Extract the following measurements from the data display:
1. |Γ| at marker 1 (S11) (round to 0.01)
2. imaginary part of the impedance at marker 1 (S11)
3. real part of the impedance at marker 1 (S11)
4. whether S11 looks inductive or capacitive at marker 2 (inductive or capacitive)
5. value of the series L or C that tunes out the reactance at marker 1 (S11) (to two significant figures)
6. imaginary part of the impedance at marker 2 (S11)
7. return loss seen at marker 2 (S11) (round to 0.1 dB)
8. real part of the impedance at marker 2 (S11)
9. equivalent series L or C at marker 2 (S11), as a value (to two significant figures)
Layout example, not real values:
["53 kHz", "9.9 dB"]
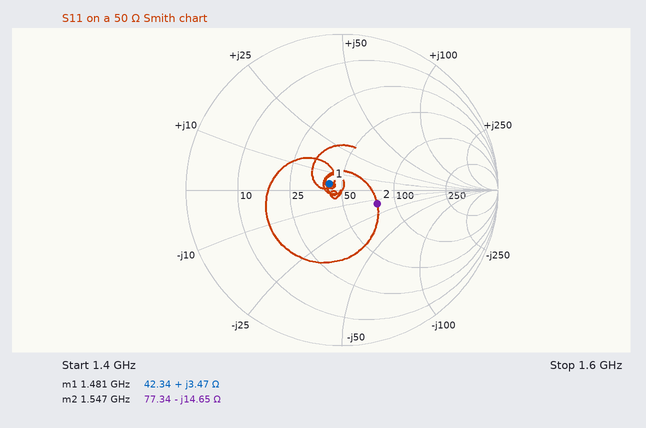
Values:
["0.09", "+3.47 Ω", "42.34 Ω", "capacitive", "31 pF", "-14.65 Ω", "12.3 dB", "77.34 Ω", "7.0 pF"]
